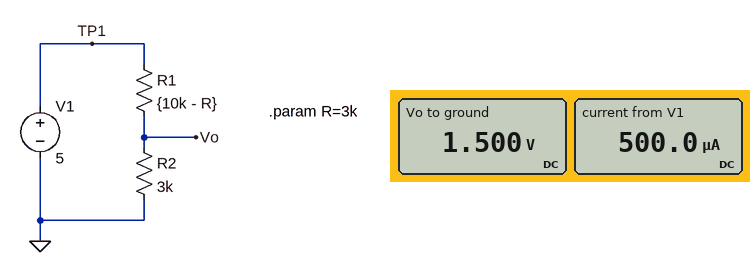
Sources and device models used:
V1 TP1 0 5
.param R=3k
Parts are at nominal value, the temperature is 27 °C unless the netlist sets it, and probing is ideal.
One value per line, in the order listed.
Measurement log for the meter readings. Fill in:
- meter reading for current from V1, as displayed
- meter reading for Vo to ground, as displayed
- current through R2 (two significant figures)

500.0 µA
1.500 V
500 µA
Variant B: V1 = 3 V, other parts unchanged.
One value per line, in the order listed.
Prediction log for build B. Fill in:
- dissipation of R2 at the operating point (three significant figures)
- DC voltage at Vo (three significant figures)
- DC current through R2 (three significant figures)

270 µW
900 mV
300 µA
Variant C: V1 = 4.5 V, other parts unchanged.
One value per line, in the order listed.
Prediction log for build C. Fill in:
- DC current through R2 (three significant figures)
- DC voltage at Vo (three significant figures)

450 µA
1.35 V
